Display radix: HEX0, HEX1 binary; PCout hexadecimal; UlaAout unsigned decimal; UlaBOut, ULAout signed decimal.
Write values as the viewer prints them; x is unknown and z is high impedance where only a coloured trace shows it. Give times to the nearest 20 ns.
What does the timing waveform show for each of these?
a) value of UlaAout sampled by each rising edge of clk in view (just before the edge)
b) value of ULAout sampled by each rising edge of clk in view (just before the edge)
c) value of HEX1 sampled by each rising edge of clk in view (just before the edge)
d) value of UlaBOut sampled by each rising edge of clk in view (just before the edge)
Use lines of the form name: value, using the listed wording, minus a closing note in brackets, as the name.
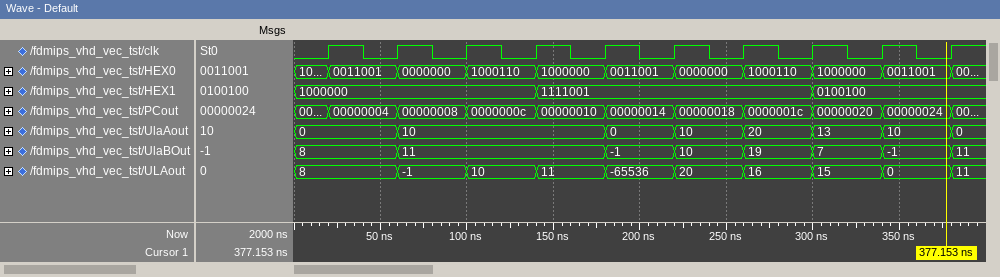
value of UlaAout sampled by each rising edge of clk in view: 0, 0, 10, 10, 10, 0, 10, 20, 13, 10
value of ULAout sampled by each rising edge of clk in view: 8, 8, -1, 10, 11, -65536, 20, 16, 15, 0
value of HEX1 sampled by each rising edge of clk in view: 1000000, 1000000, 1000000, 1000000, 1111001, 1111001, 1111001, 1111001, 0100100, 0100100
value of UlaBOut sampled by each rising edge of clk in view: 8, 8, 11, 11, 11, -1, 10, 19, 7, -1
